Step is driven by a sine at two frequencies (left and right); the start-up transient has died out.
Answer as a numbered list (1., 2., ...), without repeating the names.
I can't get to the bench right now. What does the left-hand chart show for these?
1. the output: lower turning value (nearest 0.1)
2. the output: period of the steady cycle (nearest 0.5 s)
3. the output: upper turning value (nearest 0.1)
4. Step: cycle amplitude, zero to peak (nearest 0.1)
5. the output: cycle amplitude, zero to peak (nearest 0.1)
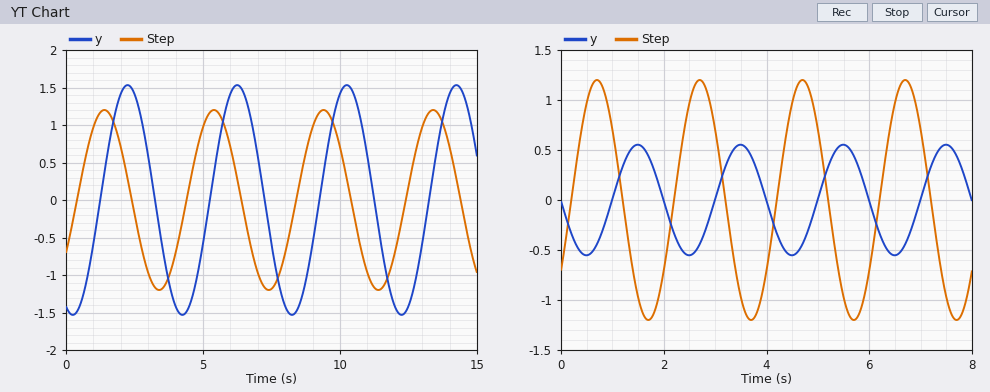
1. -1.5
2. 4.0 s
3. 1.5
4. 1.2
5. 1.5
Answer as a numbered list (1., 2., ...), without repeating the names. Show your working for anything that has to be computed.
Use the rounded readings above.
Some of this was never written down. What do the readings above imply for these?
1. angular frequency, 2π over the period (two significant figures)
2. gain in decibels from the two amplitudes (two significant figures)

1. 2π / 4 = 1.6 rad/s
2. 20 log10(1.5 / 1.2) = 1.9 dB
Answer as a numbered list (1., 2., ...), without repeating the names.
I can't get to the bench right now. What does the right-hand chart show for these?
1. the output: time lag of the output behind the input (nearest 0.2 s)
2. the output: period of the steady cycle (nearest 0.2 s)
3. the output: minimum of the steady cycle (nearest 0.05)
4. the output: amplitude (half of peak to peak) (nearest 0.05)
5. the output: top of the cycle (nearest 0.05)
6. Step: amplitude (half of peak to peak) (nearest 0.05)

1. 0.8 s
2. 2.0 s
3. -0.55
4. 0.55
5. 0.55
6. 1.20
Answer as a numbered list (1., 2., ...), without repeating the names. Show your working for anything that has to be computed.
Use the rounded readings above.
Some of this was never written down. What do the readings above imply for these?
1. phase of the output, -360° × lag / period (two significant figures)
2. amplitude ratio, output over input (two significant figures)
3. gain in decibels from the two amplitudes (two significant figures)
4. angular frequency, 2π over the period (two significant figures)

1. -360 × 0.8 / 2 = -140°
2. 0.55 / 1.2 = 0.46
3. 20 log10(0.55 / 1.2) = -6.8 dB
4. 2π / 2 = 3.1 rad/s
